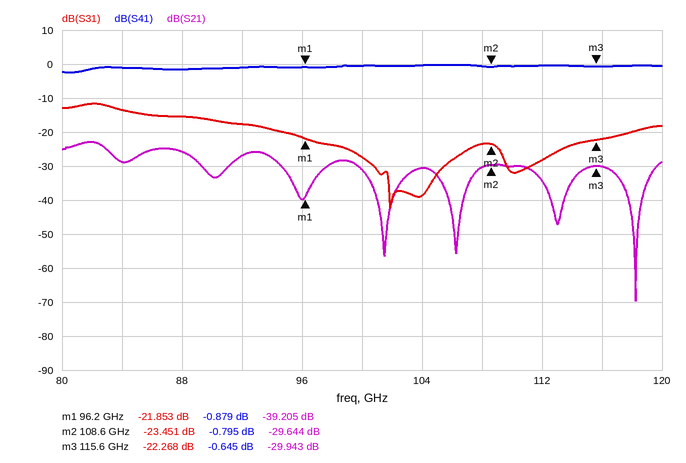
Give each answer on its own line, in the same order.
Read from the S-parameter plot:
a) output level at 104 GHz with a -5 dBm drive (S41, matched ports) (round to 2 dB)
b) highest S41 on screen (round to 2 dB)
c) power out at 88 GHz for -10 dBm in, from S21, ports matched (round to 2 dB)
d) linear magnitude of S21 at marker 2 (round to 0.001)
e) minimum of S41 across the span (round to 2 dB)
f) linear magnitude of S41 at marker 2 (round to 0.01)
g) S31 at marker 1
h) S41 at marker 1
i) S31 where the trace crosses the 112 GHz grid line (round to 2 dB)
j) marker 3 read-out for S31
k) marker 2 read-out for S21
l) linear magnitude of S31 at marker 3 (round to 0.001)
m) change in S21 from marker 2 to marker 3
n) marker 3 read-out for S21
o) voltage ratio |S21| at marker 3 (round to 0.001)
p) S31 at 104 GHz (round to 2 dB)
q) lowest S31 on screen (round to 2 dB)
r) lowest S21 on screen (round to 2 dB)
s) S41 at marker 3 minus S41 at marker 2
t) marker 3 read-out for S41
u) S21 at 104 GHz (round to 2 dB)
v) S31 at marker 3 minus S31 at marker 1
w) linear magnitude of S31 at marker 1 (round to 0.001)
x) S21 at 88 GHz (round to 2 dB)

-6 dBm
0 dB
-36 dBm
0.033
-2 dB
0.91
-21.853 dB
-0.879 dB
-28 dB
-22.268 dB
-29.644 dB
0.077
-0.299 dB
-29.943 dB
0.032
-38 dB
-42 dB
-70 dB
0.150 dB
-0.645 dB
-30 dB
-0.415 dB
0.081
-26 dB
